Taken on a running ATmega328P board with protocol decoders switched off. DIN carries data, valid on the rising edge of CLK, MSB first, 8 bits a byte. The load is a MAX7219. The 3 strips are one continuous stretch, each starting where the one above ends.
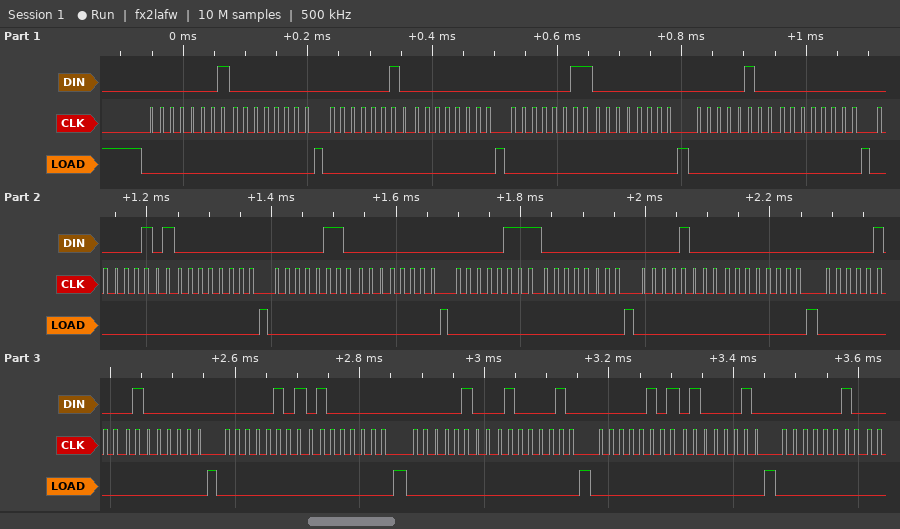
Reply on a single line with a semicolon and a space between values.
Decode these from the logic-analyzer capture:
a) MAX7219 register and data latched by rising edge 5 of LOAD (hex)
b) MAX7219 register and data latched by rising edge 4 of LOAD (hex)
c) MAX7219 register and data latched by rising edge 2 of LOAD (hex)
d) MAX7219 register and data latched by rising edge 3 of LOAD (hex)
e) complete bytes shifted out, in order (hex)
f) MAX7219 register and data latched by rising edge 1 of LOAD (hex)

register 0x5, data 0x00; register 0x4, data 0x00; register 0x2, data 0x00; register 0x3, data 0x00; 0x01 0x00 0x02 0x00 0x03 0x00 0x04 0x00 0x05 0x00 0x06 0x00 0x07 0x00 0x08 0x00 0x04 0x40 0x05 0x40 0x04 0x42 0x05 0x42 0x02; register 0x1, data 0x00
